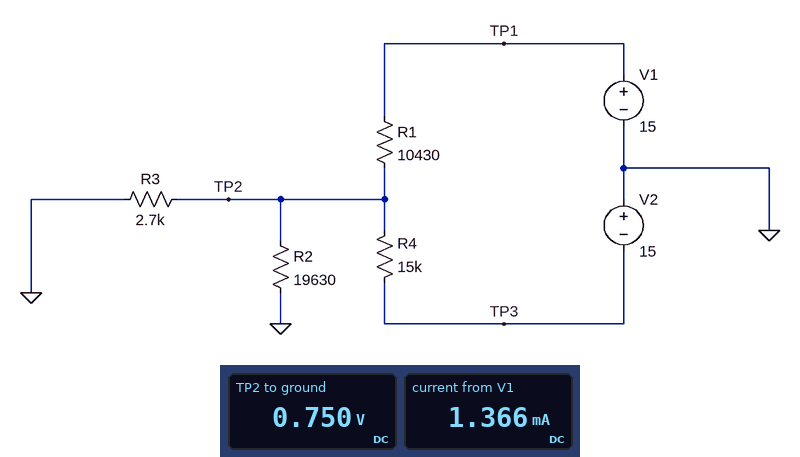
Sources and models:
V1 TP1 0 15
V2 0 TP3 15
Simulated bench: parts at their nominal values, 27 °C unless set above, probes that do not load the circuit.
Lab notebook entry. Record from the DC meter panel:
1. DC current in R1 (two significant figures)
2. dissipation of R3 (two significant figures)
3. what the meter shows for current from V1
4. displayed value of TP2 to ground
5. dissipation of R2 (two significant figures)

1.4 mA
210 µW
1.366 mA
0.750 V
29 µW
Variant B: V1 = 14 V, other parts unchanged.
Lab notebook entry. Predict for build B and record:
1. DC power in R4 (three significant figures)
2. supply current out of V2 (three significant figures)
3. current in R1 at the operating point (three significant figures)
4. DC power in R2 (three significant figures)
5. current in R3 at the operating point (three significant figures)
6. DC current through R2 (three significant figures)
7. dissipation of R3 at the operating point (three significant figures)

16.2 mW
1.04 mA
1.29 mA
17.5 µW
217 µA
29.9 µA
127 µW
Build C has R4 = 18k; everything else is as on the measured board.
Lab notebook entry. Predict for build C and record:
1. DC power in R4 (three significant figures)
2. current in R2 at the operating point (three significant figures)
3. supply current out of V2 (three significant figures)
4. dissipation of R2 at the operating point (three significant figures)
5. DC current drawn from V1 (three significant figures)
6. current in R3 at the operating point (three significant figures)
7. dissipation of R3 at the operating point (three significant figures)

14.3 mW
53.8 µA
892 µA
56.8 µW
1.34 mA
391 µA
413 µW
